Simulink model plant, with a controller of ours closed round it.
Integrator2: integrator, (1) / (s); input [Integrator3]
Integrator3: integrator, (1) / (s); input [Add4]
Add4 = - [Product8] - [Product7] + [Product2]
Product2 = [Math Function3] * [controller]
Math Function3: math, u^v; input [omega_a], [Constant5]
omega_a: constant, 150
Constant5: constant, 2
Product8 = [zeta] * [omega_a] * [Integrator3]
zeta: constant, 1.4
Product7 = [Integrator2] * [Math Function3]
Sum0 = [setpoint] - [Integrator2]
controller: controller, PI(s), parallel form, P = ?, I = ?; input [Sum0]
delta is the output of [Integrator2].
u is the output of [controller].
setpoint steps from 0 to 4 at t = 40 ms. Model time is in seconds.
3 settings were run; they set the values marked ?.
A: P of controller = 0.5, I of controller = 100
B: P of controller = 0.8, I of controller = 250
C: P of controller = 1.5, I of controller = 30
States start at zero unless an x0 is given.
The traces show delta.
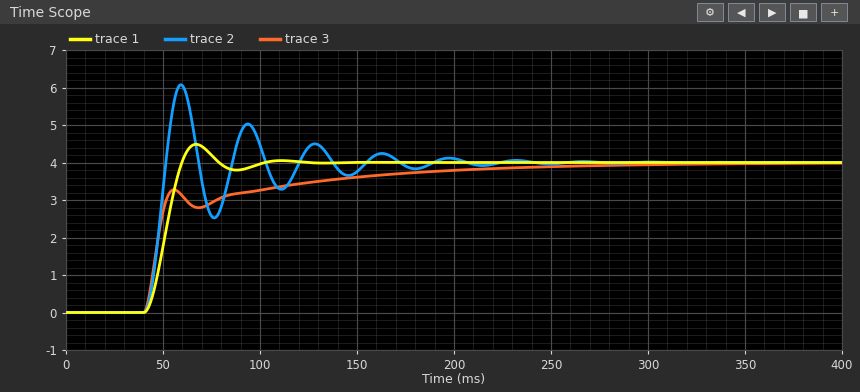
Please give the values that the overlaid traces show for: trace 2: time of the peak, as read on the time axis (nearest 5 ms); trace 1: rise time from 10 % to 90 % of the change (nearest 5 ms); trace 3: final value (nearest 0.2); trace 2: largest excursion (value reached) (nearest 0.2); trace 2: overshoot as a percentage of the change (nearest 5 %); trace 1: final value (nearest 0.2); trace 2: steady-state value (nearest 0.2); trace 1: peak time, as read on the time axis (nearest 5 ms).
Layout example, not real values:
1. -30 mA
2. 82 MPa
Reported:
1. 60 ms
2. 15 ms
3. 4.0
4. 6.0
5. 50 %
6. 4.0
7. 4.0
8. 65 ms
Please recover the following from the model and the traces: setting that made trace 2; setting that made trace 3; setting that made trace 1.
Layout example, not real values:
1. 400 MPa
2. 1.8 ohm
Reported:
1. B
2. C
3. A
